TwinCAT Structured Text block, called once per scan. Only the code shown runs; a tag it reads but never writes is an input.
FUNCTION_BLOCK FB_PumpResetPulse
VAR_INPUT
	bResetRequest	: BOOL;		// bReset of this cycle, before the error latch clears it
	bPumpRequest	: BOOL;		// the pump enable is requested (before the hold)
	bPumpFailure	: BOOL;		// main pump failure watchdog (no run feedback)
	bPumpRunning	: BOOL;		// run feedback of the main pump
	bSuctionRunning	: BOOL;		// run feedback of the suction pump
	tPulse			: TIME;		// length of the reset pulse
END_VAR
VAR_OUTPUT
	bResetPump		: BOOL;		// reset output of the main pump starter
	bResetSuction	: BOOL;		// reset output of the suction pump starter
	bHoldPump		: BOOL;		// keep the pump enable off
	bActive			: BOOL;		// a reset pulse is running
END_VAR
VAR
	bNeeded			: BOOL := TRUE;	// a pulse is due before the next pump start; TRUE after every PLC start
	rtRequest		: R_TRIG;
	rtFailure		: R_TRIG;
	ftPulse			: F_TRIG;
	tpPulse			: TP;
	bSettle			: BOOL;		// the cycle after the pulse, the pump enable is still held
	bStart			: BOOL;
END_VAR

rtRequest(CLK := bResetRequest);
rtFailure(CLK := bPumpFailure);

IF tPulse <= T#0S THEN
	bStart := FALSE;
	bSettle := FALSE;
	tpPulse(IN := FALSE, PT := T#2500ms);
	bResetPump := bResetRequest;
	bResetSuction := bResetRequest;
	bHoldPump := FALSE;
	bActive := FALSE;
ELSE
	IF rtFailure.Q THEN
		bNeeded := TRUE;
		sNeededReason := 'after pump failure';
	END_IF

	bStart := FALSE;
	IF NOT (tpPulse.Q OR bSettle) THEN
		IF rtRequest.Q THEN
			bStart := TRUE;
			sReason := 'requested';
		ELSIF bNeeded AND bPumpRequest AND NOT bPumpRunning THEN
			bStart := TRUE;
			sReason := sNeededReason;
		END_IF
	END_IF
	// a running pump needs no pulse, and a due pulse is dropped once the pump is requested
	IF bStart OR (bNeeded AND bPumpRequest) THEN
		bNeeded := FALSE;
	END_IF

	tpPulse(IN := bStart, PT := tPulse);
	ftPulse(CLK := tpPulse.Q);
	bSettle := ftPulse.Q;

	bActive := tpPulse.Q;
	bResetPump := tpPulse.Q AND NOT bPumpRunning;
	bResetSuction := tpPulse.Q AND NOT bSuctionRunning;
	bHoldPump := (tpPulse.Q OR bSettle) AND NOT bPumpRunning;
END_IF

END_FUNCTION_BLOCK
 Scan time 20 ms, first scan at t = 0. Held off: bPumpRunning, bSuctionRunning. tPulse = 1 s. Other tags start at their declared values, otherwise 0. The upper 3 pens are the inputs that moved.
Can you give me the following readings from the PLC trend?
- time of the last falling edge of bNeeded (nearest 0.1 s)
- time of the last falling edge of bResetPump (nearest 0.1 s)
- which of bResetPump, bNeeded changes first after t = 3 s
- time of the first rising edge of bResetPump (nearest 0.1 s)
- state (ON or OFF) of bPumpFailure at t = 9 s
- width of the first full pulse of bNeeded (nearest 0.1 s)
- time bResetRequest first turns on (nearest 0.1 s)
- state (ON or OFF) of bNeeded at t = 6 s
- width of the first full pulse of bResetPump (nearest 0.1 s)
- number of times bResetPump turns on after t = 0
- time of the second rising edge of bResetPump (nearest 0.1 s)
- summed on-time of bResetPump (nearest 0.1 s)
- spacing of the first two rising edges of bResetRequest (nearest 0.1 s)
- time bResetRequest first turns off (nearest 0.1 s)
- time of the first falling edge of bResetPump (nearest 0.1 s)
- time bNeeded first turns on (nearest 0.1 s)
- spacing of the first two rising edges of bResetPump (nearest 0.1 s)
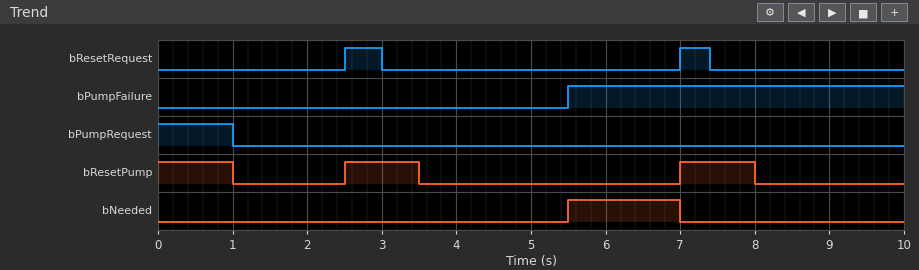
7.0 s
8.0 s
bResetPump
2.5 s
ON
1.5 s
2.5 s
ON
1.0 s
2
7.0 s
3.0 s
4.5 s
3.0 s
1.0 s
5.5 s
4.5 s
